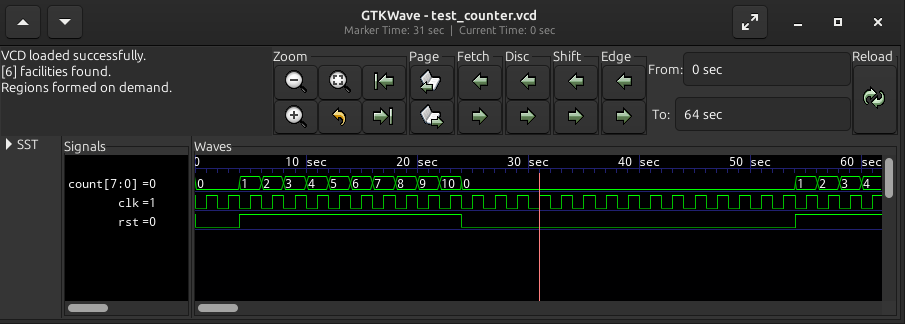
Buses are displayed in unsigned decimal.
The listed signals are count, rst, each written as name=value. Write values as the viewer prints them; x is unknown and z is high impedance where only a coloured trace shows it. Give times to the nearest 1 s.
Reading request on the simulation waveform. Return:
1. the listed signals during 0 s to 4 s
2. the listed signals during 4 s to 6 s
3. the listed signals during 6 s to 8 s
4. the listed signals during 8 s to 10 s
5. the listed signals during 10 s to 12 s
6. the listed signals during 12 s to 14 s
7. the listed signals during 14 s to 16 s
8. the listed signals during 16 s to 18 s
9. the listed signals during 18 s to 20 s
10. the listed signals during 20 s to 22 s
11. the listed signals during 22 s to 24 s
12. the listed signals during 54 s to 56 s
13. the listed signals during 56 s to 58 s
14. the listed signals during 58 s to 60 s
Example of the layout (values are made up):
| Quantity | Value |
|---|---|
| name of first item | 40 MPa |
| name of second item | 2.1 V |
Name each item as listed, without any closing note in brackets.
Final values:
| Quantity | Value |
|---|---|
| the listed signals during 0 s to 4 s | count=0, rst=0 |
| the listed signals during 4 s to 6 s | count=1, rst=1 |
| the listed signals during 6 s to 8 s | count=2, rst=1 |
| the listed signals during 8 s to 10 s | count=3, rst=1 |
| the listed signals during 10 s to 12 s | count=4, rst=1 |
| the listed signals during 12 s to 14 s | count=5, rst=1 |
| the listed signals during 14 s to 16 s | count=6, rst=1 |
| the listed signals during 16 s to 18 s | count=7, rst=1 |
| the listed signals during 18 s to 20 s | count=8, rst=1 |
| the listed signals during 20 s to 22 s | count=9, rst=1 |
| the listed signals during 22 s to 24 s | count=10, rst=1 |
| the listed signals during 54 s to 56 s | count=1, rst=1 |
| the listed signals during 56 s to 58 s | count=2, rst=1 |
| the listed signals during 58 s to 60 s | count=3, rst=1 |
